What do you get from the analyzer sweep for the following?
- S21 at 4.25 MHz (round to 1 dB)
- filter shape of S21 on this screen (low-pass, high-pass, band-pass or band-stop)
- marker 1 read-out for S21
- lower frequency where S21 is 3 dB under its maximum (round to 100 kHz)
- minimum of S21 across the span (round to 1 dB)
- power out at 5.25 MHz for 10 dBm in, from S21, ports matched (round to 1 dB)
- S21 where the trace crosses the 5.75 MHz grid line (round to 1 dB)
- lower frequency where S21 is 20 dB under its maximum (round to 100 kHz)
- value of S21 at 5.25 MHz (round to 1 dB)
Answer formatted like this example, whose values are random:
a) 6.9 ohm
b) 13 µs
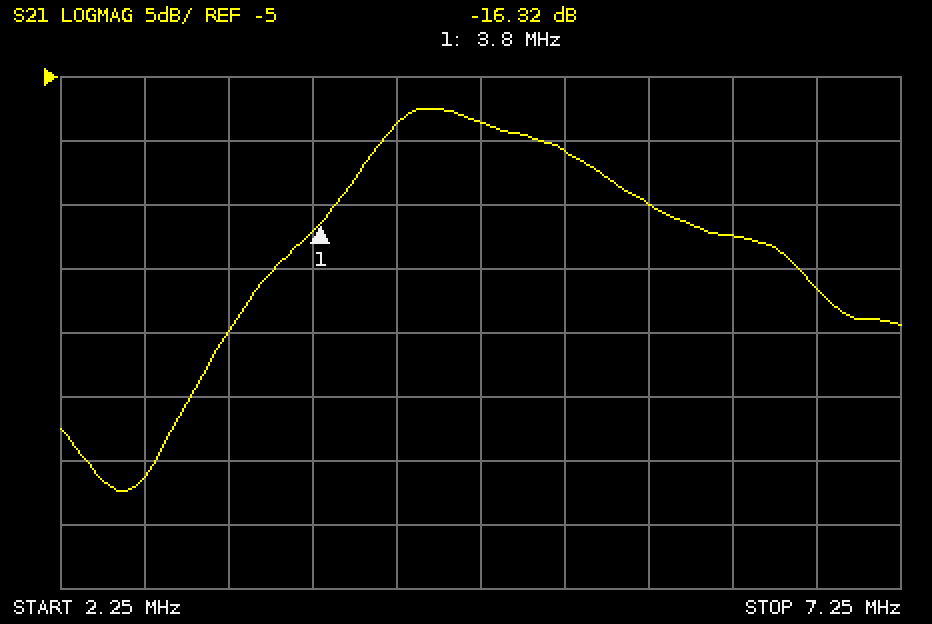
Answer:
a) -9 dB
b) band-pass
c) -16.32 dB
d) 4.1 MHz
e) -37 dB
f) -1 dBm
g) -15 dB
h) 3.1 MHz
i) -11 dB
